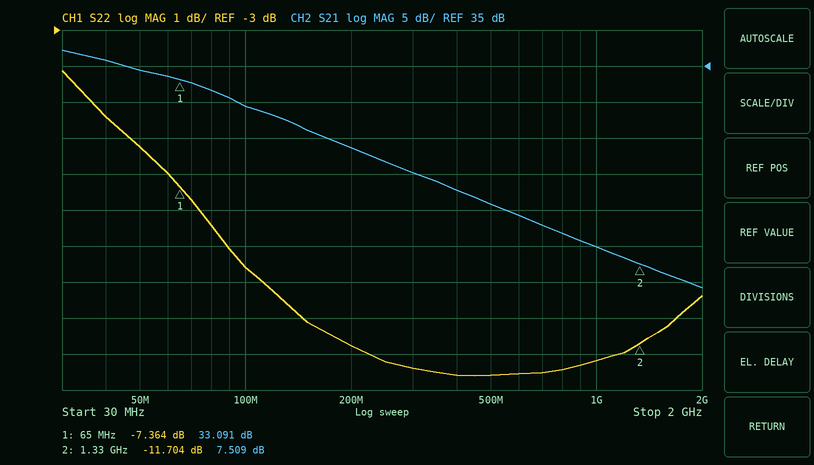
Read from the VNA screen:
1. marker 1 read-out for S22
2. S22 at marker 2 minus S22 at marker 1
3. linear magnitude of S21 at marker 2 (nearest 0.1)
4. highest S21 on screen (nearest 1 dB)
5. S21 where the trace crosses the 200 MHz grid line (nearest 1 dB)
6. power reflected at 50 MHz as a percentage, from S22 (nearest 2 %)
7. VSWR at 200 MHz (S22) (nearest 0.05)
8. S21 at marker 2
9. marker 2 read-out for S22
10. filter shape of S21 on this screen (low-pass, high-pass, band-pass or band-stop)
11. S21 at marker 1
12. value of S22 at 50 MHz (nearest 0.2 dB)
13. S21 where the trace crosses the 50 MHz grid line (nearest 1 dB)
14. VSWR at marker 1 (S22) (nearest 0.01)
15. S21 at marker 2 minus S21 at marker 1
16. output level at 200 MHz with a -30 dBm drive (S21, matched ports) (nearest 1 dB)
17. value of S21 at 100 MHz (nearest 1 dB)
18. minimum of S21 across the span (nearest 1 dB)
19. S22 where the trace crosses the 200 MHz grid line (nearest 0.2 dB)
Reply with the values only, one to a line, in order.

-7.364 dB
-4.340 dB
2.4
37 dB
24 dB
24 %
1.70
7.509 dB
-11.704 dB
low-pass
33.091 dB
-6.2 dB
34 dB
2.50
-25.582 dB
-6 dBm
29 dB
4 dB
-11.8 dB
